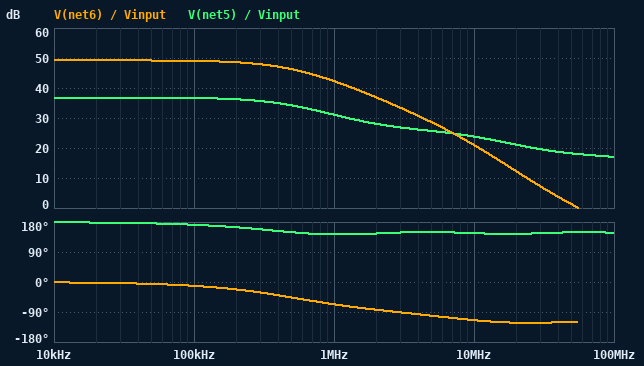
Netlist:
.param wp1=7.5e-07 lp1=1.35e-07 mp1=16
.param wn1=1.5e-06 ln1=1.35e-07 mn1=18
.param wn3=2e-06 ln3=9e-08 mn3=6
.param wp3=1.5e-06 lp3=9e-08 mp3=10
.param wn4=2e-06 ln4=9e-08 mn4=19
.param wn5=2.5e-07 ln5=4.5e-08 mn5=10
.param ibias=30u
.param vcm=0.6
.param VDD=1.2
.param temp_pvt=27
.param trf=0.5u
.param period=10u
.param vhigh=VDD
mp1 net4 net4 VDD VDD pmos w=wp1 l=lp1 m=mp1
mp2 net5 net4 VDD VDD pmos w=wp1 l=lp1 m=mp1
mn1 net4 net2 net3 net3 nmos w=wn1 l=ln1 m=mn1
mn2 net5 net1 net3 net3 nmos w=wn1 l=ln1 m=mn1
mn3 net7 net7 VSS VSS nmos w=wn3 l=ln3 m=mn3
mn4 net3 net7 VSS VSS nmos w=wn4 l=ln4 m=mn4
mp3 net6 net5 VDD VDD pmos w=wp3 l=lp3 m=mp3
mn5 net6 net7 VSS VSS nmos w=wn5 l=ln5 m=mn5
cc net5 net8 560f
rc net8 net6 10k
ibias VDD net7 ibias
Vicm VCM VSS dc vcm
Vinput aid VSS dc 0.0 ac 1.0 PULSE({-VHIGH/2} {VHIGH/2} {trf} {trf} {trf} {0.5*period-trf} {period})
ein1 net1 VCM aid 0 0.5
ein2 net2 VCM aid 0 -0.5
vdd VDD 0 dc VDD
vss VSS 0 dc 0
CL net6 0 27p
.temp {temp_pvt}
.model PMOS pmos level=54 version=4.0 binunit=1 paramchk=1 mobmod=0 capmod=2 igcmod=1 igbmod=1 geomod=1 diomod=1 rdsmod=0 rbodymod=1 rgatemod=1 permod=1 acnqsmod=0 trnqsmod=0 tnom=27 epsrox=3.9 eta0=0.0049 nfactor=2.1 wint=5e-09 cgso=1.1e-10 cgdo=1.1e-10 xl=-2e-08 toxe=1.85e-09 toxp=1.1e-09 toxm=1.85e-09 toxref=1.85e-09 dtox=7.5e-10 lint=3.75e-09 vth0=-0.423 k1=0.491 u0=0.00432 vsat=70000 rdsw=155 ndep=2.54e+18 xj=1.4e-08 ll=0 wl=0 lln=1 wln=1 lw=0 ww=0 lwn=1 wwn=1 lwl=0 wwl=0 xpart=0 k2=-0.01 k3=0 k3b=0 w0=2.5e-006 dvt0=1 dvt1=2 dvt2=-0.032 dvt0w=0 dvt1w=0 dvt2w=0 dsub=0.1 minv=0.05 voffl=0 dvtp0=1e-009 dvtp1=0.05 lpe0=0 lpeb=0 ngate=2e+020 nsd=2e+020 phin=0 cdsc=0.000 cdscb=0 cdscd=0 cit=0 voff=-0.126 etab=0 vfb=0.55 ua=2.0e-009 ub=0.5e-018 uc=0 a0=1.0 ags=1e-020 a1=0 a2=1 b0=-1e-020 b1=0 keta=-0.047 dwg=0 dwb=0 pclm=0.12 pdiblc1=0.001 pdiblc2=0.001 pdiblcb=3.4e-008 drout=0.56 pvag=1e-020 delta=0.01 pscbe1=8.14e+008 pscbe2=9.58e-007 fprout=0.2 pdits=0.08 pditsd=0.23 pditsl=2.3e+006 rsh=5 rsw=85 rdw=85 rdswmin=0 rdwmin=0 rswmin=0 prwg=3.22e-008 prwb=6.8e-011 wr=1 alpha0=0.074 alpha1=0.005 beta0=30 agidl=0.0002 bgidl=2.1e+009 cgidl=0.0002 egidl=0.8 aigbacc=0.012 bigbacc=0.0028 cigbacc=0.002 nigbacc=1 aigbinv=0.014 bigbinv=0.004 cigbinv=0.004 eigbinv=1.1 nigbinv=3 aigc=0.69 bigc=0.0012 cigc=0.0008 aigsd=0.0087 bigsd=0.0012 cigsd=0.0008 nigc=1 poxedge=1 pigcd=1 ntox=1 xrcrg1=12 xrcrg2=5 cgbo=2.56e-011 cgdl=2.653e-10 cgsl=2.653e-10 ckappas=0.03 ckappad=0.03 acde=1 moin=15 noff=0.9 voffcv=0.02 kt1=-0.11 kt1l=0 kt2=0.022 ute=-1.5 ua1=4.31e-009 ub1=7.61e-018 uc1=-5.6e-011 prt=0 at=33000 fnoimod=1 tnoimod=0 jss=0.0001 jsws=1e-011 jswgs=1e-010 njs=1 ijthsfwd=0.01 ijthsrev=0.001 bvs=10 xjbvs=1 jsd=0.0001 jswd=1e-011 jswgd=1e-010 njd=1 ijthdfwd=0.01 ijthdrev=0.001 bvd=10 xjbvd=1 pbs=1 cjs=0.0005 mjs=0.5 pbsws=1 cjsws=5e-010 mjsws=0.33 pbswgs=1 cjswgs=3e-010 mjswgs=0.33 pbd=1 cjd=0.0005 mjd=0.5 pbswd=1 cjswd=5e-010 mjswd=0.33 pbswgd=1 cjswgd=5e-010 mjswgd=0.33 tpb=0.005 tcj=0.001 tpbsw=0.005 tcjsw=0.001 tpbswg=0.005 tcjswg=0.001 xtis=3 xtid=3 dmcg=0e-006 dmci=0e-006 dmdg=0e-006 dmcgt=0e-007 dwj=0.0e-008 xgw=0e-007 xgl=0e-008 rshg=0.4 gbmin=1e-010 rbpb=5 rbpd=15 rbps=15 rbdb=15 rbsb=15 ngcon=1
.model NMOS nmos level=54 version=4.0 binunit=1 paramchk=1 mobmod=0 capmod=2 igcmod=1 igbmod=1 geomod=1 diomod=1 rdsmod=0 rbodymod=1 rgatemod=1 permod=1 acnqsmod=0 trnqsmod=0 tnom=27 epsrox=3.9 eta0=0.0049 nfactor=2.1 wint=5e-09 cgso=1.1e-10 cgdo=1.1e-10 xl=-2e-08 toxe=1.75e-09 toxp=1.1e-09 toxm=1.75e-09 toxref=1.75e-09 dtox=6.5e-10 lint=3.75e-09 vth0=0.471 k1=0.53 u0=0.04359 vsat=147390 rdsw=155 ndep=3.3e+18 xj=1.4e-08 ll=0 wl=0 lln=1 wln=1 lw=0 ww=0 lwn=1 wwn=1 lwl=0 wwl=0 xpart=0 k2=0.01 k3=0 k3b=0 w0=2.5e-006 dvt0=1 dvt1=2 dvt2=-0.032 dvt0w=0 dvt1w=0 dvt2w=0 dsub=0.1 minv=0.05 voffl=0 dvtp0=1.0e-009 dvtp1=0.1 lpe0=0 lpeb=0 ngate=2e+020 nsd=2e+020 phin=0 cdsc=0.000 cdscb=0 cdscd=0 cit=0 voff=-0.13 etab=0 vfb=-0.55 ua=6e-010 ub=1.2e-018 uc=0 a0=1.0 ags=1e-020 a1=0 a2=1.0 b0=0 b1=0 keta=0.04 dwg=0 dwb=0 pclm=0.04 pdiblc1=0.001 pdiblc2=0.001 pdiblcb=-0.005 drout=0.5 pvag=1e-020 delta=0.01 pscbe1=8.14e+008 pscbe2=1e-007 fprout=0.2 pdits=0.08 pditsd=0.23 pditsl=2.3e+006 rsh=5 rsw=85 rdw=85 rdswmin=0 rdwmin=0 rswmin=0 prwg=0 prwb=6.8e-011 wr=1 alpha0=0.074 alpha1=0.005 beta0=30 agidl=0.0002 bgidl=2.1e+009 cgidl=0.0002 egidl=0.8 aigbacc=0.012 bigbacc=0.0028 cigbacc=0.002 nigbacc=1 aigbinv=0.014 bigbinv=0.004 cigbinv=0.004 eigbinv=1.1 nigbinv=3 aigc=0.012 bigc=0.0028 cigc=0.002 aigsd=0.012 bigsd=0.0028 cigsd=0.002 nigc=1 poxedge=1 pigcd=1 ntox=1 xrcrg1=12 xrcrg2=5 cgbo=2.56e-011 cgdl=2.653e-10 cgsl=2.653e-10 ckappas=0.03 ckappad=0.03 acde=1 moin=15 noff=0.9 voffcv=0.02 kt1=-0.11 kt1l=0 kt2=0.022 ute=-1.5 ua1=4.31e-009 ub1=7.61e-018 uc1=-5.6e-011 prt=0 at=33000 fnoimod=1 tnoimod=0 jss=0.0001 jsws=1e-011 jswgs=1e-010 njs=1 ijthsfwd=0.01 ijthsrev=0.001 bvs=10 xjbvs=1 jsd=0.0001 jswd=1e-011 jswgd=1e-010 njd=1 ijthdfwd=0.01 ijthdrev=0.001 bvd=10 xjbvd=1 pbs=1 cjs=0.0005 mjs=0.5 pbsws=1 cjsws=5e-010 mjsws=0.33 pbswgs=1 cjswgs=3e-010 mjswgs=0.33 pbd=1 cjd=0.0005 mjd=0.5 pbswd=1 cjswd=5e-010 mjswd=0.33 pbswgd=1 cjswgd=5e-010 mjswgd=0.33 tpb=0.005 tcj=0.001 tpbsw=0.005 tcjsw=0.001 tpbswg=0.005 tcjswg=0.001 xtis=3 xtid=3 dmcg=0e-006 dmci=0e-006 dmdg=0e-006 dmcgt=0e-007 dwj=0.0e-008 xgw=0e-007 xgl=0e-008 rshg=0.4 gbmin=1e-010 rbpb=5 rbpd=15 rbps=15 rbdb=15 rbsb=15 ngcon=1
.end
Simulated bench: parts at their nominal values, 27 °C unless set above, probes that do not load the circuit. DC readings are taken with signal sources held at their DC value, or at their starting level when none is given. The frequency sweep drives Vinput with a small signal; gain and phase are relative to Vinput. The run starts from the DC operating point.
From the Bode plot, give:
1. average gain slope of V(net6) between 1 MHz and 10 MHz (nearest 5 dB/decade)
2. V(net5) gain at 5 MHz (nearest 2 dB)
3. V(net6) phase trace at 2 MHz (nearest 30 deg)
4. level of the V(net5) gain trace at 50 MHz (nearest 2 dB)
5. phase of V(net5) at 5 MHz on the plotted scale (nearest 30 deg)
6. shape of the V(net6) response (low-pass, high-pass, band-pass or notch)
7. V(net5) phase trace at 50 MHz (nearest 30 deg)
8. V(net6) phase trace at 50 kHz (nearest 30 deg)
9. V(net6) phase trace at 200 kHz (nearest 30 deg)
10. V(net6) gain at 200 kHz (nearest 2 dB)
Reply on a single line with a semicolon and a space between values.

-20 dB/decade; 26 dB; -90 deg; 18 dB; 150 deg; low-pass; 150 deg; 0 deg; -30 deg; 48 dB
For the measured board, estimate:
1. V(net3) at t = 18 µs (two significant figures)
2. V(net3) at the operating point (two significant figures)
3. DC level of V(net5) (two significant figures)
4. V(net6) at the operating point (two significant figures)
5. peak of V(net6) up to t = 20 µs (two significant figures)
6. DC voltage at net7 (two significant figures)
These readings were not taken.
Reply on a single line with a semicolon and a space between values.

470 mV; 210 mV; 660 mV; 580 mV; 1.1 V; 380 mV
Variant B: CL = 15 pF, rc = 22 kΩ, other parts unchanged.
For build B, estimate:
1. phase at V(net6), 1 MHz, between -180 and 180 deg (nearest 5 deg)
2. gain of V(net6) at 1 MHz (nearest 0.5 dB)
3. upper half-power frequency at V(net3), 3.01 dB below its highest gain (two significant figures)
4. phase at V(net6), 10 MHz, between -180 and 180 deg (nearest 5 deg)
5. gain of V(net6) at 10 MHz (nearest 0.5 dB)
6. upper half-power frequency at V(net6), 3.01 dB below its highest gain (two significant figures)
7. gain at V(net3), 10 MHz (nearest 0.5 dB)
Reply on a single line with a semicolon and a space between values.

-60 deg; 43.0 dB; 570 kHz; -85 deg; 24.5 dB; 560 kHz; -26.0 dB
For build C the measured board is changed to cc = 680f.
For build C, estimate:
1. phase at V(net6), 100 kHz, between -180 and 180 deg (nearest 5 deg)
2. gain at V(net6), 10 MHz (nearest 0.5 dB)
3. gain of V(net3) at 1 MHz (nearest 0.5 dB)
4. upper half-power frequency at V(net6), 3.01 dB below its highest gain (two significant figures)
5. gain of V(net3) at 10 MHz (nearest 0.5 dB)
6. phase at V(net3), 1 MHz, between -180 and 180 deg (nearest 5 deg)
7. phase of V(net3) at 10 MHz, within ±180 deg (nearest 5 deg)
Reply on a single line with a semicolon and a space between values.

-15 deg; 20.0 dB; -18.5 dB; 440 kHz; -26.0 dB; 140 deg; 155 deg
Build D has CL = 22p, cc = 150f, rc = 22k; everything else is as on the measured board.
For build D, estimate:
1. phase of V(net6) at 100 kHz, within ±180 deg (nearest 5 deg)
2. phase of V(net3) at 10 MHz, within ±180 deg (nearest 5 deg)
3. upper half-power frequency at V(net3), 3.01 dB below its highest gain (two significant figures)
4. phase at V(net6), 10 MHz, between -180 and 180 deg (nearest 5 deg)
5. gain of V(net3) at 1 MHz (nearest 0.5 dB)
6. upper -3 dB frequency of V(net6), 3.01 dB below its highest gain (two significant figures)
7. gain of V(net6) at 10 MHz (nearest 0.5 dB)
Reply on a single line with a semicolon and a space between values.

-5 deg; 155 deg; 1.9 MHz; -110 deg; -13.0 dB; 1.2 MHz; 29.5 dB
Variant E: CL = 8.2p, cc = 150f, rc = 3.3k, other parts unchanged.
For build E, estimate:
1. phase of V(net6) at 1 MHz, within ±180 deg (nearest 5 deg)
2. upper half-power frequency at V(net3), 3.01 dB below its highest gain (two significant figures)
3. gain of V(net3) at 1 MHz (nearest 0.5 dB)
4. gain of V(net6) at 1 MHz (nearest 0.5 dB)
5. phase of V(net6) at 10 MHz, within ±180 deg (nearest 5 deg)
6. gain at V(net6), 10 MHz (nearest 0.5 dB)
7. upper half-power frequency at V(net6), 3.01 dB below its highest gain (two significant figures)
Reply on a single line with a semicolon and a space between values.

-30 deg; 2.0 MHz; -12.5 dB; 48.0 dB; -95 deg; 33.5 dB; 1.8 MHz
